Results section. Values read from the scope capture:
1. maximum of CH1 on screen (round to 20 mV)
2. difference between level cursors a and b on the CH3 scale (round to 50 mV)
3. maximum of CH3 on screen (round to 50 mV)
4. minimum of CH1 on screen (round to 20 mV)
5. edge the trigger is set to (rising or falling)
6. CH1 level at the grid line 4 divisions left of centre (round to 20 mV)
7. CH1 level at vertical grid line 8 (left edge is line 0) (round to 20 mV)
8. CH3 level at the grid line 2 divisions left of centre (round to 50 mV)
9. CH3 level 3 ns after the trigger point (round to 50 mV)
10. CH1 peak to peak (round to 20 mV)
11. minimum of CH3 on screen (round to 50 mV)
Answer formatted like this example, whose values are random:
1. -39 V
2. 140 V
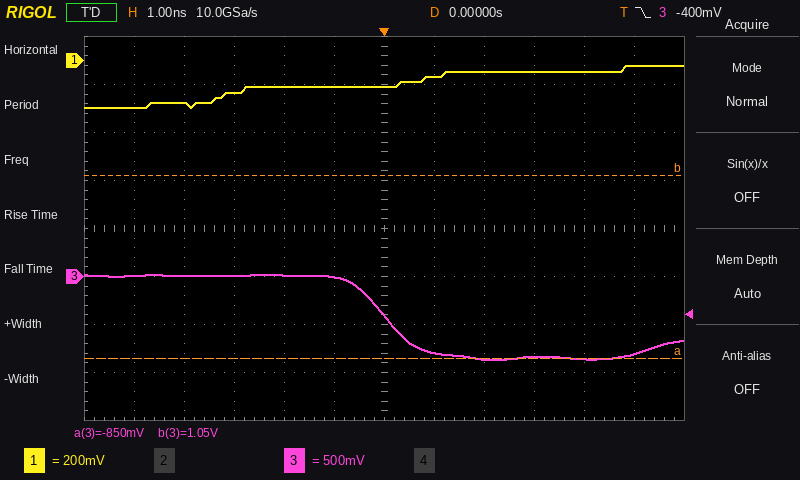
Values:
1. -20 mV
2. 1.90 V
3. 0 mV
4. -200 mV
5. falling
6. -180 mV
7. -40 mV
8. 0 mV
9. -850 mV
10. 180 mV
11. -850 mV
